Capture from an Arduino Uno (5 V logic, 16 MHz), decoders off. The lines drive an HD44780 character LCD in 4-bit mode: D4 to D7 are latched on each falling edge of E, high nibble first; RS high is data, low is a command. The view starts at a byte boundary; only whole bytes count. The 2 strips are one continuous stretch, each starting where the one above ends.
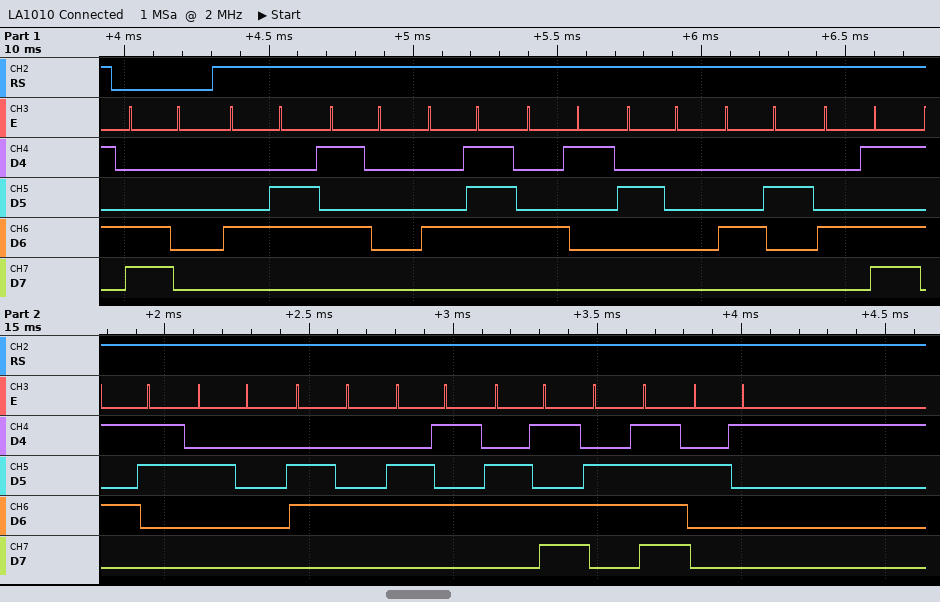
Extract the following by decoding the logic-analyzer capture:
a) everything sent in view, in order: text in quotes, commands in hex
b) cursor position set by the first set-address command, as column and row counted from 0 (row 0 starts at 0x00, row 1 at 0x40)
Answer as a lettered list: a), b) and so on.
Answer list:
a) 0xC0 "FPGA BMS demo!"
b) column 0, row 1
